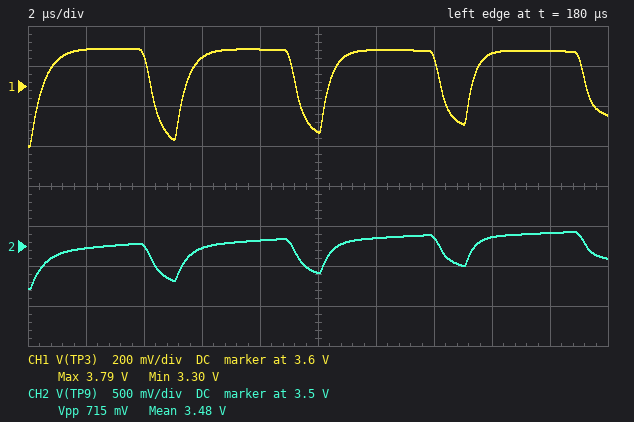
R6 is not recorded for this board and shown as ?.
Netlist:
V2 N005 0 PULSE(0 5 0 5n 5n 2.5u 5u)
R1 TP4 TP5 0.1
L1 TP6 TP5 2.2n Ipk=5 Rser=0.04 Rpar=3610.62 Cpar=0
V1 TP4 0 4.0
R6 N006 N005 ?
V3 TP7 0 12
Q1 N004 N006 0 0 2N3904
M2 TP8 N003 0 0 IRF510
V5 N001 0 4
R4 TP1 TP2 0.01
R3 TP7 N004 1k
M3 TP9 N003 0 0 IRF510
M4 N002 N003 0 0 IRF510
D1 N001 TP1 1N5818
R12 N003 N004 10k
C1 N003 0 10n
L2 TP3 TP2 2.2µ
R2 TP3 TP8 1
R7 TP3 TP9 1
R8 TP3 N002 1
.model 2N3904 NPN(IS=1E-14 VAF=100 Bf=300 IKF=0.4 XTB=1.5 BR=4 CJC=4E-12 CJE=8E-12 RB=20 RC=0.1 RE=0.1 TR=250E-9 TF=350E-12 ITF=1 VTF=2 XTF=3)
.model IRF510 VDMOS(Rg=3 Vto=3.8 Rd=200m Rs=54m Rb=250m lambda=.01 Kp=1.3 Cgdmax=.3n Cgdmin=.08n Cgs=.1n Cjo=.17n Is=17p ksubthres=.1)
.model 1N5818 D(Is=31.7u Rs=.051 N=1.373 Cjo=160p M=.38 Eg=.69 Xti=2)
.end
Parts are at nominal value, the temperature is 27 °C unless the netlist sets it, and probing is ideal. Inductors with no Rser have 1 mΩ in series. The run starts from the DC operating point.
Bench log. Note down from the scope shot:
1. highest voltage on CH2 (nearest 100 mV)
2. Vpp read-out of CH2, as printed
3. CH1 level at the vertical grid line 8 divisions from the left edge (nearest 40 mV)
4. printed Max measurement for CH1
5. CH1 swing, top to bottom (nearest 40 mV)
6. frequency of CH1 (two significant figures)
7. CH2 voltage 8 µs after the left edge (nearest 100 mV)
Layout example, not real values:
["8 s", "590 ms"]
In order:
["3.7 V", "715 mV", "3.76 V", "3.79 V", "480 mV", "200 kHz", "3.6 V"]
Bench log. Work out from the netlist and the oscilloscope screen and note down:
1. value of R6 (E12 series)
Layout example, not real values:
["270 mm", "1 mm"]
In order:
["12 kΩ"]
